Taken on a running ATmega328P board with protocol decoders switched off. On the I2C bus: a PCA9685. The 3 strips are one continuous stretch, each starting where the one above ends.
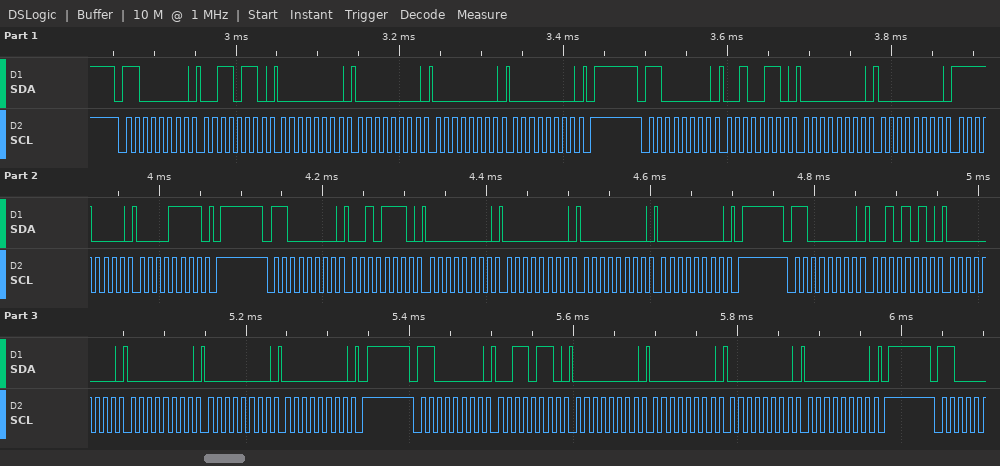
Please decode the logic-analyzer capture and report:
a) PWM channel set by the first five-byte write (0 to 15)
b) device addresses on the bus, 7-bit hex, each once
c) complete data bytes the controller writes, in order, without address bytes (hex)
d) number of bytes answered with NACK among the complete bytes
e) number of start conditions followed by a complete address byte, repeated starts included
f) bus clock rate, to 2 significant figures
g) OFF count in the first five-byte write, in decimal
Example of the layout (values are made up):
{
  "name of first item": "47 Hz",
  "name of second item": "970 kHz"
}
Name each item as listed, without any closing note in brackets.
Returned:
{
  "PWM channel set by the first five-byte write": "12",
  "device addresses on the bus, 7-bit hex, each once": "0x60",
  "complete data bytes the controller writes, in order, without address bytes": "36 00 00 00 00 26 00 00 F0 0F 2E 00 00 00 00 2A 00 00 00 00 36 00 00 00 00",
  "number of bytes answered with NACK among the complete bytes": "0",
  "number of start conditions followed by a complete address byte, repeated starts included": "5",
  "bus clock rate, to 2 significant figures": "100 kHz",
  "OFF count in the first five-byte write, in decimal": "0"
}
